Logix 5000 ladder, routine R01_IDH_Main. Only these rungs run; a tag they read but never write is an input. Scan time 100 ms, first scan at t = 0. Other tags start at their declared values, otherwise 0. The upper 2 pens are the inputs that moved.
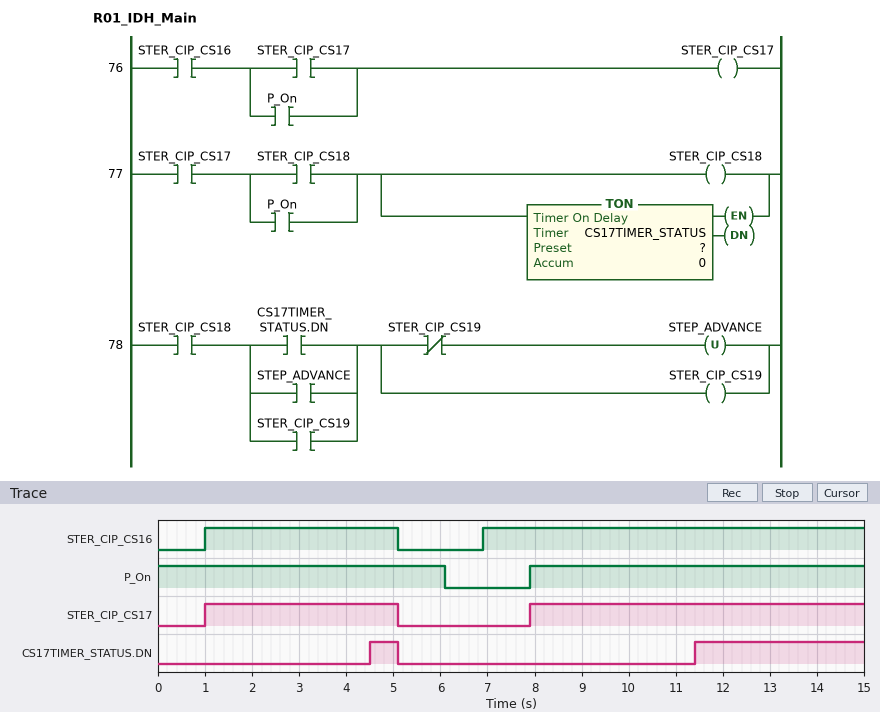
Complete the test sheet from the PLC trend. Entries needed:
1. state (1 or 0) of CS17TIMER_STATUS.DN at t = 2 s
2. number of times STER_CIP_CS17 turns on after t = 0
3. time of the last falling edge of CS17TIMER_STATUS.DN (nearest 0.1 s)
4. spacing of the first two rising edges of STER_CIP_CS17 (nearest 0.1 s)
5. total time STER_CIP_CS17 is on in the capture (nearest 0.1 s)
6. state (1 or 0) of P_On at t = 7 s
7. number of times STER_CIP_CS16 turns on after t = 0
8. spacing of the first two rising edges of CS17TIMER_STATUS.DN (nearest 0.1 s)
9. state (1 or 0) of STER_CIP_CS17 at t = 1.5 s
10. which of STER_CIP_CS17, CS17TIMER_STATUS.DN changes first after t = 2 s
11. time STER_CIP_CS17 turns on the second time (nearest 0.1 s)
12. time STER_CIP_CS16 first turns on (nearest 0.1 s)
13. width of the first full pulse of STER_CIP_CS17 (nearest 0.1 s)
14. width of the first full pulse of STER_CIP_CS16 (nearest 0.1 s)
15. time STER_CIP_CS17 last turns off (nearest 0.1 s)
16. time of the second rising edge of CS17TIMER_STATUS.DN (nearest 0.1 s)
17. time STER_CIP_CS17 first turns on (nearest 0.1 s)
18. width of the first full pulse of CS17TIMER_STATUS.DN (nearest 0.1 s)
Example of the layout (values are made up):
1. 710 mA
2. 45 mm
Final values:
1. 0
2. 2
3. 5.1 s
4. 6.9 s
5. 11.2 s
6. 0
7. 2
8. 6.9 s
9. 1
10. CS17TIMER_STATUS.DN
11. 7.9 s
12. 1.0 s
13. 4.1 s
14. 4.1 s
15. 5.1 s
16. 11.4 s
17. 1.0 s
18. 0.6 s
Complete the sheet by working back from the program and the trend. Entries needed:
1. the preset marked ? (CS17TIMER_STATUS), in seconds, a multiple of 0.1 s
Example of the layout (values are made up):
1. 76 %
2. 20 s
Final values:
1. 3.5 s
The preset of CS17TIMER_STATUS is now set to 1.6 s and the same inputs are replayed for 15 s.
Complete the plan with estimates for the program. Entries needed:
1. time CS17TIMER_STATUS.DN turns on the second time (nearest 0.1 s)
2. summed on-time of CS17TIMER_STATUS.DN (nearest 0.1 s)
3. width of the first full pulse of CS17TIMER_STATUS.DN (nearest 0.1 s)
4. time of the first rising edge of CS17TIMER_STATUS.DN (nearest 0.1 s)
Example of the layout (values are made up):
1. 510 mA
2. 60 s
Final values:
1. 9.5 s
2. 8.0 s
3. 2.5 s
4. 2.6 s
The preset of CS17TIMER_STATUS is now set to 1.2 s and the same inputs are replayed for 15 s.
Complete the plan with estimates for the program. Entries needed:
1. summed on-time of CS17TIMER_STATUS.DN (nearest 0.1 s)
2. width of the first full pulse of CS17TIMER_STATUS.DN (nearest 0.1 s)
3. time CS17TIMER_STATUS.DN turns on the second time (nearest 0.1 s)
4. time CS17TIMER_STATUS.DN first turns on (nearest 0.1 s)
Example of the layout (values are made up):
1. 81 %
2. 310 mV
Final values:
1. 8.8 s
2. 2.9 s
3. 9.1 s
4. 2.2 s
